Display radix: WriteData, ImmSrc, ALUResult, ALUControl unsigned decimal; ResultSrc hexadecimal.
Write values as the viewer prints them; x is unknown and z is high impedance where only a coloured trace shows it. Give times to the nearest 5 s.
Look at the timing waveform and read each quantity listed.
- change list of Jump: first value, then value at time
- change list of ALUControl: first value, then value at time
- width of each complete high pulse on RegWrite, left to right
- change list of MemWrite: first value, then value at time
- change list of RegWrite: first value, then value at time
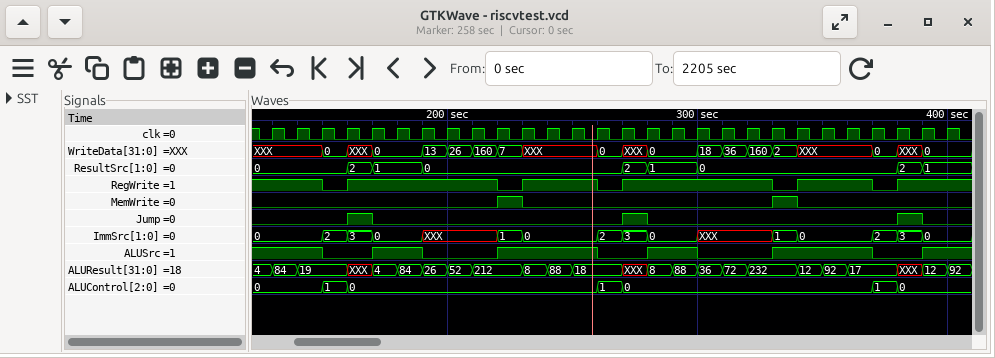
0, 1 at 160 s, 0 at 170 s, 1 at 270 s, 0 at 280 s, 1 at 380 s, 0 at 390 s
0, 1 at 150 s, 0 at 160 s, 1 at 260 s, 0 at 270 s, 1 at 370 s, 0 at 380 s
60 s, 30 s, 60 s, 30 s
0, 1 at 220 s, 0 at 230 s, 1 at 330 s, 0 at 340 s
1, 0 at 150 s, 1 at 160 s, 0 at 220 s, 1 at 230 s, 0 at 260 s, 1 at 270 s, 0 at 330 s, 1 at 340 s, 0 at 370 s, 1 at 380 s
